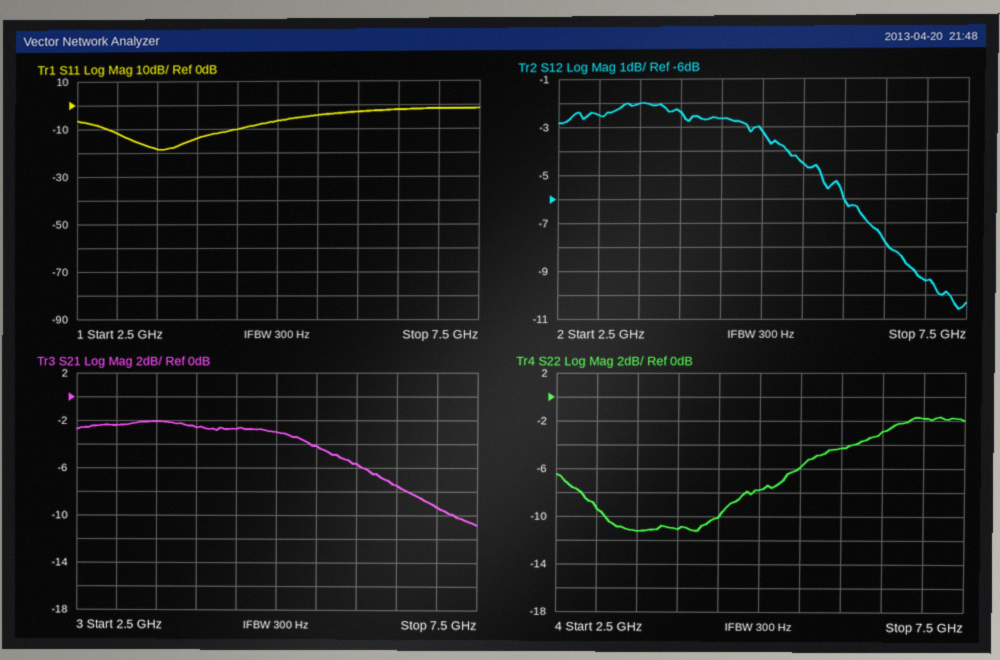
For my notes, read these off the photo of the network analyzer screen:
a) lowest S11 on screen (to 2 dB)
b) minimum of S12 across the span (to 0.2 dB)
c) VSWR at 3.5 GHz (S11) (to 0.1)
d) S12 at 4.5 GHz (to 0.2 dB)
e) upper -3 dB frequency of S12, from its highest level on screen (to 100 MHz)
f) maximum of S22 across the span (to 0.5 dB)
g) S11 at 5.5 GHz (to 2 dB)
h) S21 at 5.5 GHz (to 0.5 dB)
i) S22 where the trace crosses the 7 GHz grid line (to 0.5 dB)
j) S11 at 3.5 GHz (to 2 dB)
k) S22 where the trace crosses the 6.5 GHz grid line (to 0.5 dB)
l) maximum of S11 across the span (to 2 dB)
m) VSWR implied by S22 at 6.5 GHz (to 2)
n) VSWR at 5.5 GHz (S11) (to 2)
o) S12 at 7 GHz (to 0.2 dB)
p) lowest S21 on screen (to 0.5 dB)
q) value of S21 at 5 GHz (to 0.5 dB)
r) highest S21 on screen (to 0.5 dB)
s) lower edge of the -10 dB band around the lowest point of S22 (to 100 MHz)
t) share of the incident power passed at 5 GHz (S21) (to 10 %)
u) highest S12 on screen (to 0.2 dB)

-18 dB
-10.6 dB
1.3
-2.6 dB
5.7 GHz
-1.5 dB
-4 dB
-4.0 dB
-2.0 dB
-18 dB
-3.0 dB
-2 dB
6
4
-9.4 dB
-11.0 dB
-3.0 dB
-2.0 dB
3.1 GHz
50 %
-2.0 dB
